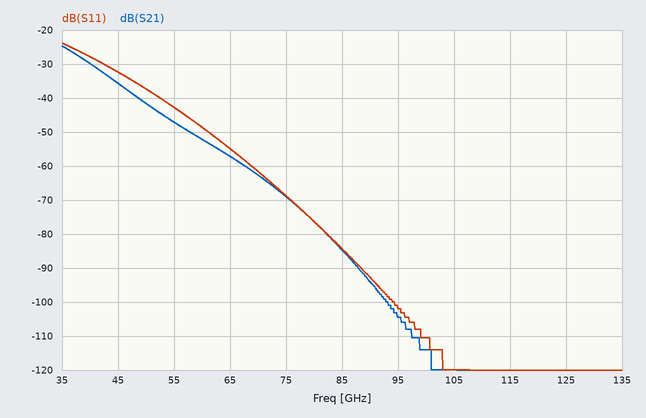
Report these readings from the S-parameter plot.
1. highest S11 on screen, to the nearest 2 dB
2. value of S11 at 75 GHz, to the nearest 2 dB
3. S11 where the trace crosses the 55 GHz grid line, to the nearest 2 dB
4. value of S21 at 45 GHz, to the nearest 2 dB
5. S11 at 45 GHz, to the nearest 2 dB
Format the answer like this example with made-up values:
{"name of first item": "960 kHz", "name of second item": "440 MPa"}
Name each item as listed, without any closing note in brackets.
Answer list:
{"highest S11 on screen, to the nearest 2 dB": "-24 dB", "value of S11 at 75 GHz, to the nearest 2 dB": "-68 dB", "S11 where the trace crosses the 55 GHz grid line, to the nearest 2 dB": "-42 dB", "value of S21 at 45 GHz, to the nearest 2 dB": "-36 dB", "S11 at 45 GHz, to the nearest 2 dB": "-32 dB"}
